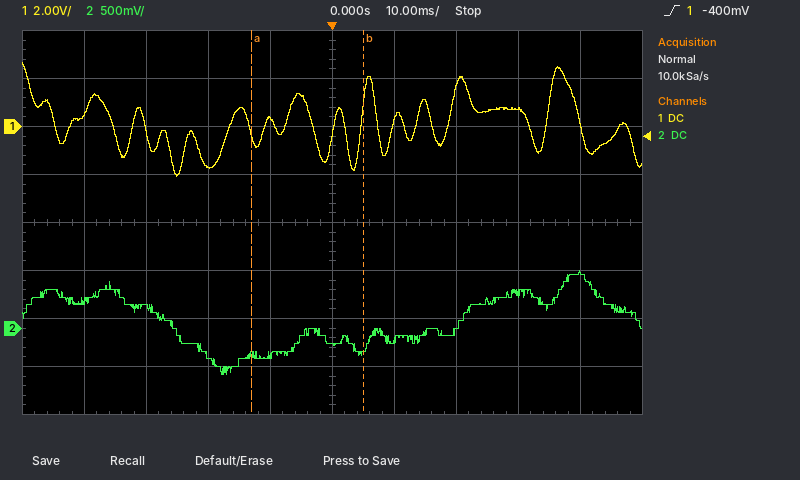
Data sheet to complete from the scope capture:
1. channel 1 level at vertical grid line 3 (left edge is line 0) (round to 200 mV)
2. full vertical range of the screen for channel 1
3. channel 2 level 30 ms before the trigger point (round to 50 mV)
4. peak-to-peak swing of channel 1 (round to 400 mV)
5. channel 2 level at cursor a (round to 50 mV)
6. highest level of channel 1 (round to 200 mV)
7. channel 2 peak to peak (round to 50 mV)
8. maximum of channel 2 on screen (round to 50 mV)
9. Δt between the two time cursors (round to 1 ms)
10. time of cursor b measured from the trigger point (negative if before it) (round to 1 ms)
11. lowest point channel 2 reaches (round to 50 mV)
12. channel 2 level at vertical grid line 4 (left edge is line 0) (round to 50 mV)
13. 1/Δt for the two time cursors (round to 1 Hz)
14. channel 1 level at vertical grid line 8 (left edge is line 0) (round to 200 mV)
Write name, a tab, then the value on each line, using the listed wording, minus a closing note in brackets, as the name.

channel 1 level at vertical grid line 3 (left edge is line 0)	-1.6 V
full vertical range of the screen for channel 1	16 V
channel 2 level 30 ms before the trigger point	200 mV
peak-to-peak swing of channel 1	4.8 V
channel 2 level at cursor a	-300 mV
highest level of channel 1	2.6 V
channel 2 peak to peak	1.10 V
maximum of channel 2 on screen	600 mV
Δt between the two time cursors	18 ms
time of cursor b measured from the trigger point (negative if before it)	+5 ms
lowest point channel 2 reaches	-500 mV
channel 2 level at vertical grid line 4 (left edge is line 0)	-300 mV
1/Δt for the two time cursors	56 Hz
channel 1 level at vertical grid line 8 (left edge is line 0)	800 mV
